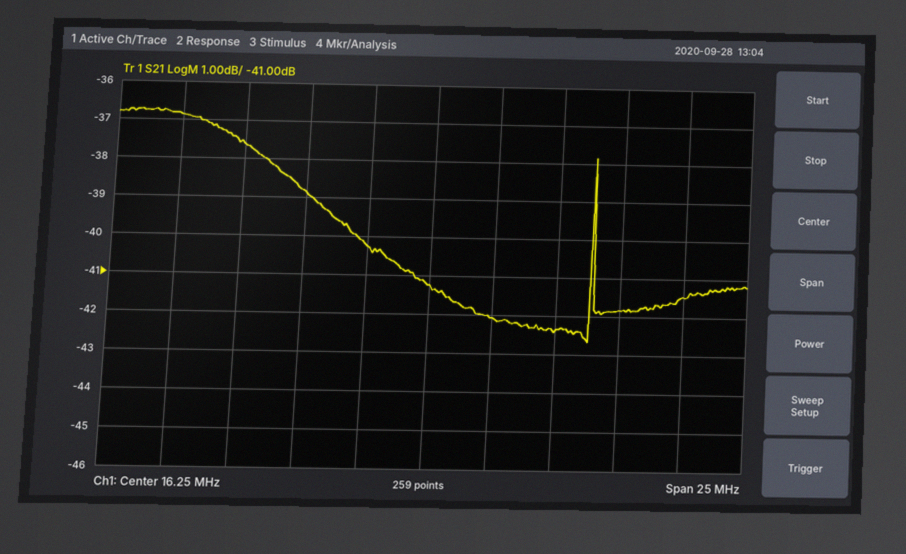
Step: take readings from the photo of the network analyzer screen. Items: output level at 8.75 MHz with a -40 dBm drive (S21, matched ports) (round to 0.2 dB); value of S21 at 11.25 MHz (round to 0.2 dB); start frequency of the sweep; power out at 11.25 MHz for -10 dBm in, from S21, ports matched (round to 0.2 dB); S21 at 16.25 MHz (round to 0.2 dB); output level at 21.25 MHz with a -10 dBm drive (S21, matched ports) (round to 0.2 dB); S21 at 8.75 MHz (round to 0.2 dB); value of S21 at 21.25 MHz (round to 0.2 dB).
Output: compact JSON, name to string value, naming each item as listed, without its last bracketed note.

{"output level at 8.75 MHz with a -40 dBm drive (S21, matched ports)": "-77.6 dBm", "value of S21 at 11.25 MHz": "-38.8 dB", "start frequency of the sweep": "3.75 MHz", "power out at 11.25 MHz for -10 dBm in, from S21, ports matched": "-48.8 dBm", "S21 at 16.25 MHz": "-41.2 dB", "output level at 21.25 MHz with a -10 dBm drive (S21, matched ports)": "-52.4 dBm", "S21 at 8.75 MHz": "-37.6 dB", "value of S21 at 21.25 MHz": "-42.4 dB"}
